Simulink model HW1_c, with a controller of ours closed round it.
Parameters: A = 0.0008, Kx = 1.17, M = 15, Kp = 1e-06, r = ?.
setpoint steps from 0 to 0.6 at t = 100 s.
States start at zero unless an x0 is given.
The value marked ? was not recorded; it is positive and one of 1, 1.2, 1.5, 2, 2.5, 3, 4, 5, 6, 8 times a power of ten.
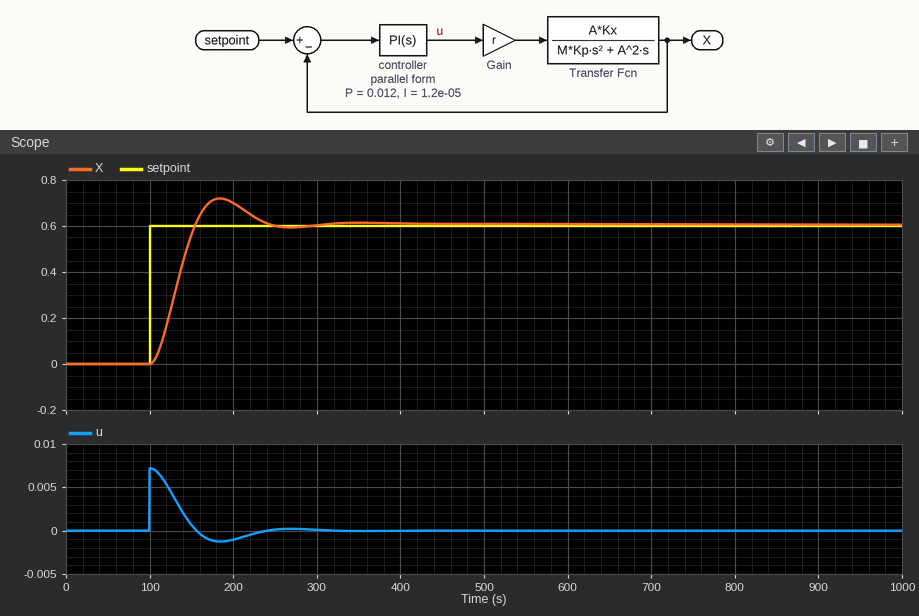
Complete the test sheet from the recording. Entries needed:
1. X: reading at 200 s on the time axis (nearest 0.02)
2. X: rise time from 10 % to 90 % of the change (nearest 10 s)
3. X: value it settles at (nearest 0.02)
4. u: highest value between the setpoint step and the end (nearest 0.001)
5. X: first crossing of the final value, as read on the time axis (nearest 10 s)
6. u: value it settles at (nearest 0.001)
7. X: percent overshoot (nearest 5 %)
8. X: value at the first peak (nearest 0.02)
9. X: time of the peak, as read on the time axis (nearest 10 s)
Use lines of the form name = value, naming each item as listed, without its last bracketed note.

X: reading at 200 s on the time axis = 0.70
X: rise time from 10 % to 90 % of the change = 40 s
X: value it settles at = 0.60
u: highest value between the setpoint step and the end = 0.007
X: first crossing of the final value, as read on the time axis = 150 s
u: value it settles at = 0.000
X: percent overshoot = 20 %
X: value at the first peak = 0.72
X: time of the peak, as read on the time axis = 180 s
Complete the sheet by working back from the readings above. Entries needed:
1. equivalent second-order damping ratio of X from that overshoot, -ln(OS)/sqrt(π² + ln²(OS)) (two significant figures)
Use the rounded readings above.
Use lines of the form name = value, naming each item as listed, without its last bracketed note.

equivalent second-order damping ratio of X from that overshoot, -ln(OS)/sqrt(π² + ln²(OS)) = 0.46
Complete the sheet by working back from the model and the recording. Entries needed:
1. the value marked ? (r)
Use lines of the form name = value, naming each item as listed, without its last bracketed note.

the value marked ? = 0.0025
